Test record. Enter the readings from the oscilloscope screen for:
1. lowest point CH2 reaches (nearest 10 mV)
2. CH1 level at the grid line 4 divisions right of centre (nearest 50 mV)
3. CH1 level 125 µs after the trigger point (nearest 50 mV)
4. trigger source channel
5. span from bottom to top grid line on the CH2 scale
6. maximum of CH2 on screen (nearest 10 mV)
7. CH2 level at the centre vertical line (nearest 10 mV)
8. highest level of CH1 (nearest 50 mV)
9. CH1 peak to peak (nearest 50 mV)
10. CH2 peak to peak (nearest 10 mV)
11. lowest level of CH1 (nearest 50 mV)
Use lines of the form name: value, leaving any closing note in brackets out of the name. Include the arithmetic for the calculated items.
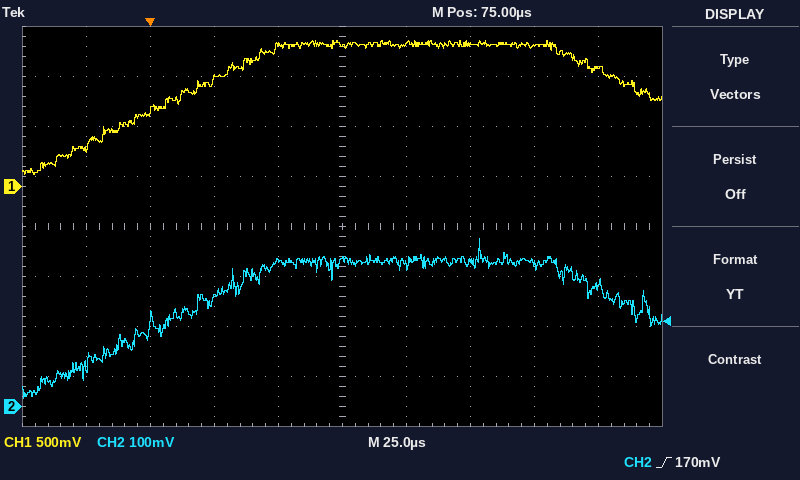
lowest point CH2 reaches: 20 mV
CH1 level at the grid line 4 divisions right of centre: 1.20 V
CH1 level 125 µs after the trigger point: 1.40 V
trigger source channel: CH2
span from bottom to top grid line on the CH2 scale: 800 mV
maximum of CH2 on screen: 340 mV
CH2 level at the centre vertical line: 290 mV
highest level of CH1: 1.45 V
CH1 peak to peak: 1.45 V − (100 mV) = 1.35 V
CH2 peak to peak: 340 mV − (20 mV) = 320 mV
lowest level of CH1: 100 mV
